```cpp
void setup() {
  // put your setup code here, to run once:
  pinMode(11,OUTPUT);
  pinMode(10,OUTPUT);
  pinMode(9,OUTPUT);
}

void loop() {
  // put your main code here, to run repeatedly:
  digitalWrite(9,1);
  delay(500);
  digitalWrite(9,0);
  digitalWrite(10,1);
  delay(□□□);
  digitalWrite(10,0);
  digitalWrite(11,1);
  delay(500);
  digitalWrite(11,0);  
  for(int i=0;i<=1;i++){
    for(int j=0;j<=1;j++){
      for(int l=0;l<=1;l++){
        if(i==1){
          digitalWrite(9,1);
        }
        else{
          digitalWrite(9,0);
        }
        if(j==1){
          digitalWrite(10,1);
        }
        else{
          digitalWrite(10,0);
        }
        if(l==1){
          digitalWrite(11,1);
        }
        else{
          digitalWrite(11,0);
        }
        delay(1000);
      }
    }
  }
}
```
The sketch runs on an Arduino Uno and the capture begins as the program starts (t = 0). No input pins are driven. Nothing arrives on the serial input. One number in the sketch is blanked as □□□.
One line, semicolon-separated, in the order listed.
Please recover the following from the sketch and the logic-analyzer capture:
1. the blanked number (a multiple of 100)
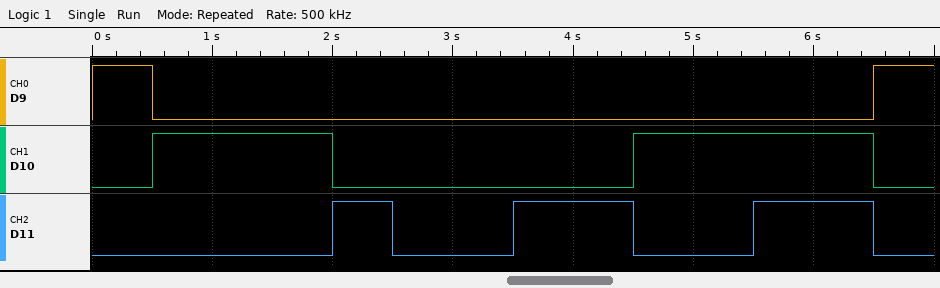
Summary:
1500
